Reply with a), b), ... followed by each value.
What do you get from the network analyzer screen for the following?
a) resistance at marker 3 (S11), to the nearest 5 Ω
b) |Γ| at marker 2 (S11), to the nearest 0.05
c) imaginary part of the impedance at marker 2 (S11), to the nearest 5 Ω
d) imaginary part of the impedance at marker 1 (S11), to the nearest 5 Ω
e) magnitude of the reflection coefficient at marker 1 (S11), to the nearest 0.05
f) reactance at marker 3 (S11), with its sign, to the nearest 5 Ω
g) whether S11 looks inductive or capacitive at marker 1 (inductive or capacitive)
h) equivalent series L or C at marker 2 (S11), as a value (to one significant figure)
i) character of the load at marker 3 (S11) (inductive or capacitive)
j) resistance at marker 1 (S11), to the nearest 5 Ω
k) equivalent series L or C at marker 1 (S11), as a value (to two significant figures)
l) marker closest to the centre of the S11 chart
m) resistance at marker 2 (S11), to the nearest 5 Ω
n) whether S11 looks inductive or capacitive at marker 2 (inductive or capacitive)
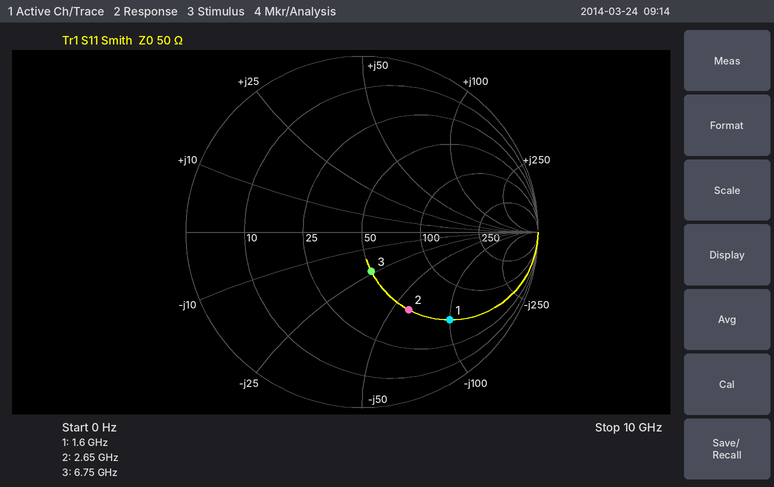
a) 50 Ω
b) 0.50
c) -60 Ω
d) -100 Ω
e) 0.70
f) -25 Ω
g) capacitive
h) 1.0 pF
i) capacitive
j) 50 Ω
k) 1.0 pF
l) marker 3
m) 50 Ω
n) capacitive
